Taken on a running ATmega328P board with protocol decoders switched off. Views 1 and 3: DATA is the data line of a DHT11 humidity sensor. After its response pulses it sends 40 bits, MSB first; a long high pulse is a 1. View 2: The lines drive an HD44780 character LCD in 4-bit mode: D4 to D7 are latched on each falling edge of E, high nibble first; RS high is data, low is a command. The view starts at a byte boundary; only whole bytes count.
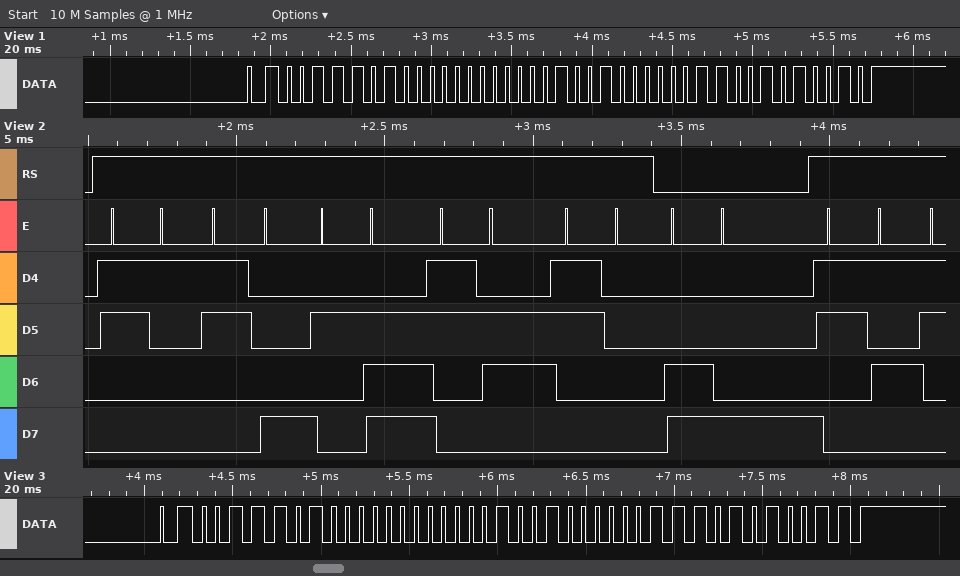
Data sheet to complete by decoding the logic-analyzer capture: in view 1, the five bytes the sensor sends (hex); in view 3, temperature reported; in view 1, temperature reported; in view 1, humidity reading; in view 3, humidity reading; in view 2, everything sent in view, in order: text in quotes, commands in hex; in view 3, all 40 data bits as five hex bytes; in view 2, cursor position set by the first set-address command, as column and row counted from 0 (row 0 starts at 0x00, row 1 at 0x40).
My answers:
3A 00 12 06 52
18.7 °C
18.6 °C
58 %
58 %
"18.60" 0xC8 "5"
3A 00 12 07 53
column 8, row 1
